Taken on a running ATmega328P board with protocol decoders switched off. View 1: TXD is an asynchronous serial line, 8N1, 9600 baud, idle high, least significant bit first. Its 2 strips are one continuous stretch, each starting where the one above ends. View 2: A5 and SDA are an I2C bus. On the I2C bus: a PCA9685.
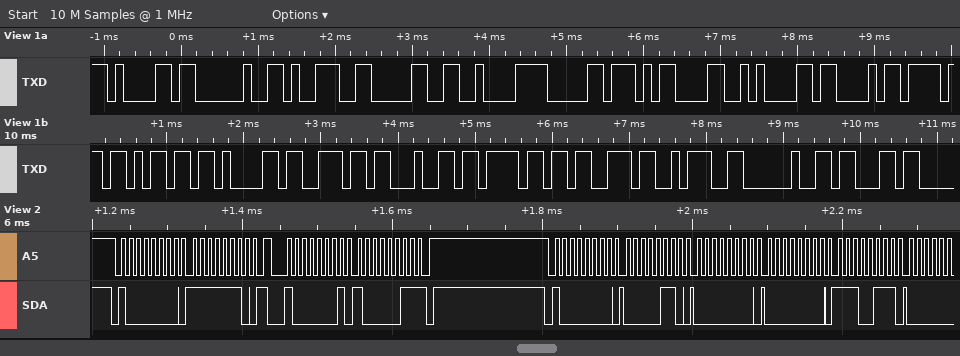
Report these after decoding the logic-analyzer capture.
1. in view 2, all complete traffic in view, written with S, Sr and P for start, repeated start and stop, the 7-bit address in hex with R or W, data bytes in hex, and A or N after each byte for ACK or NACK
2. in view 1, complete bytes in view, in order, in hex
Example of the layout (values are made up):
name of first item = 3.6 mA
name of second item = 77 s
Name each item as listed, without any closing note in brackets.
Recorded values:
in view 2, all complete traffic in view, written with S, Sr and P for start, repeated start and stop, the 7-bit address in hex with R or W, data bytes in hex, and A or N after each byte for ACK or NACK = S 40W A FE A Sr 40R A 83 N P S 40W A 06 A 00 A 00 A E7 A
in view 1, complete bytes in view, in order, in hex = 61 20 39 30 C2 B0 0D 0A 43 6F 6D 61 6E 64 6F 73 3A 20 63
